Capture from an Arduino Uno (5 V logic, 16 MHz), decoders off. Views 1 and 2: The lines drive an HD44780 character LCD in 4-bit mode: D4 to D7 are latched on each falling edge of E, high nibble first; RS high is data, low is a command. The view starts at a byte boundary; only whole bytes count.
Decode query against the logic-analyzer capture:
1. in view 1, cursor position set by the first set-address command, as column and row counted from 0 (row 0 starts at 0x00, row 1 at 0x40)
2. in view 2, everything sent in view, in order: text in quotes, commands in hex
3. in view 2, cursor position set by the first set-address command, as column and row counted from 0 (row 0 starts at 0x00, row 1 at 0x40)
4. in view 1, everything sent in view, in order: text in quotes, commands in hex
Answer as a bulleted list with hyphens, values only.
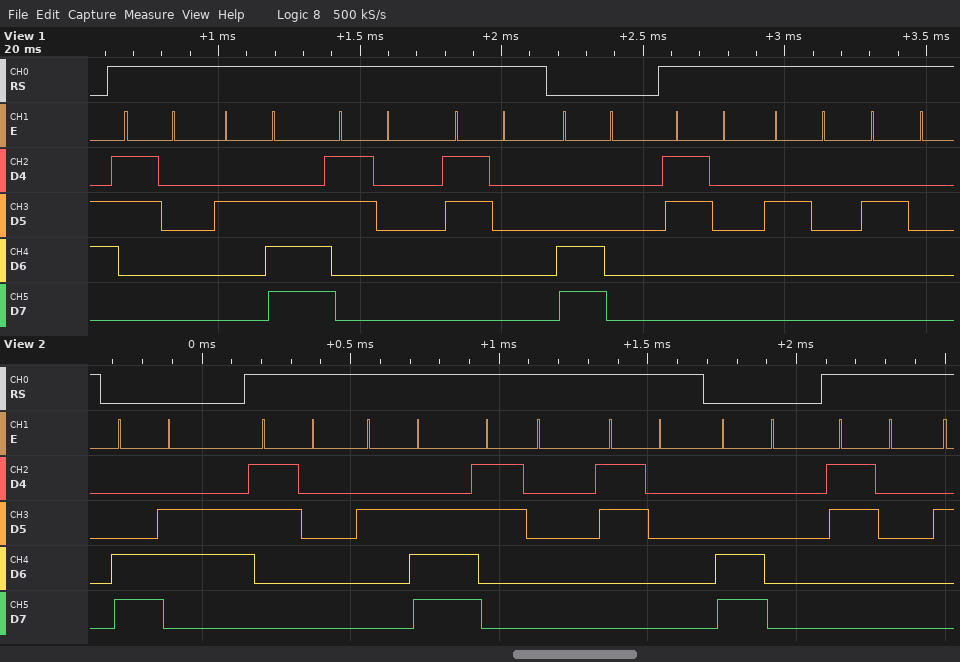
- column 0, row 1
- 0xC6 "0.00" 0xC0 "0"
- column 6, row 1
- "0.00" 0xC0 "0  "
